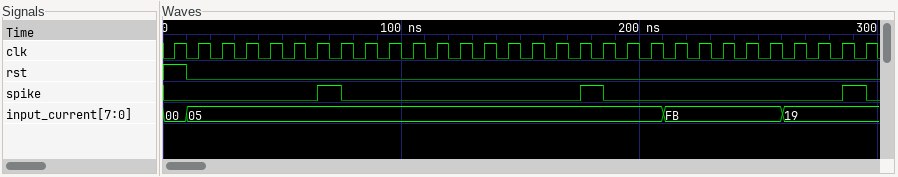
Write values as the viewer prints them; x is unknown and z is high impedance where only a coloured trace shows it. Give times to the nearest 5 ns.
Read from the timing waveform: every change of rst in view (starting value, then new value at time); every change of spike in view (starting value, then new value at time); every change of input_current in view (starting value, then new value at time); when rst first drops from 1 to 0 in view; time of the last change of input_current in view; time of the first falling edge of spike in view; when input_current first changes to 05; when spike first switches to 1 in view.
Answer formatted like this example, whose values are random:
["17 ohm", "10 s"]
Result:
["1, 0 at 10 ns", "0, 1 at 65 ns, 0 at 75 ns, 1 at 175 ns, 0 at 185 ns, 1 at 285 ns, 0 at 295 ns", "00, 05 at 10 ns, FB at 210 ns, 19 at 260 ns", "10 ns", "260 ns", "75 ns", "10 ns", "65 ns"]
